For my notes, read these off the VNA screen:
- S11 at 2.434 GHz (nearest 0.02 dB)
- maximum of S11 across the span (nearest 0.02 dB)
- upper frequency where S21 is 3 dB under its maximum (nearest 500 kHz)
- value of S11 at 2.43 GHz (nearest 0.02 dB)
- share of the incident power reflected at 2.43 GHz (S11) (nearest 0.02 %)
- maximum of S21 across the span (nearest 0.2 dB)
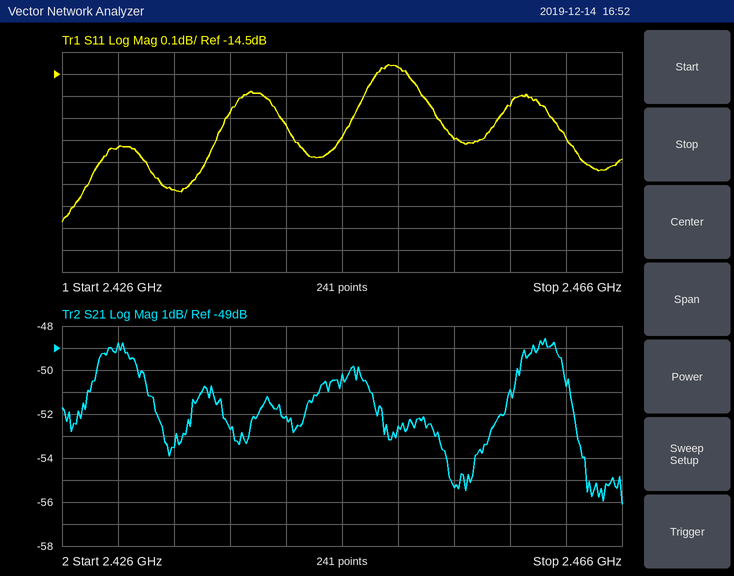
-15.02 dB
-14.46 dB
2.4625 GHz
-14.84 dB
3.28 %
-48.6 dB
